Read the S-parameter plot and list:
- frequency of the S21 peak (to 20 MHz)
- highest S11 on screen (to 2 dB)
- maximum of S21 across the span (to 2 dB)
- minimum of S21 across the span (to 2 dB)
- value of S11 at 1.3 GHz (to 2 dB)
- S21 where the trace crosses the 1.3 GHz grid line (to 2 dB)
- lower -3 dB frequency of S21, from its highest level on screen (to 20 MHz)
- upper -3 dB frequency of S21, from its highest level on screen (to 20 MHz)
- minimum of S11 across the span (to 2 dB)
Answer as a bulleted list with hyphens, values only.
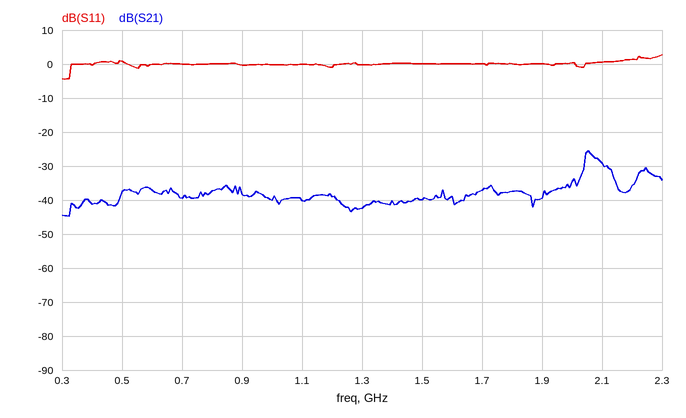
- 2.06 GHz
- 2 dB
- -26 dB
- -44 dB
- 0 dB
- -42 dB
- 2.04 GHz
- 2.10 GHz
- -4 dB
